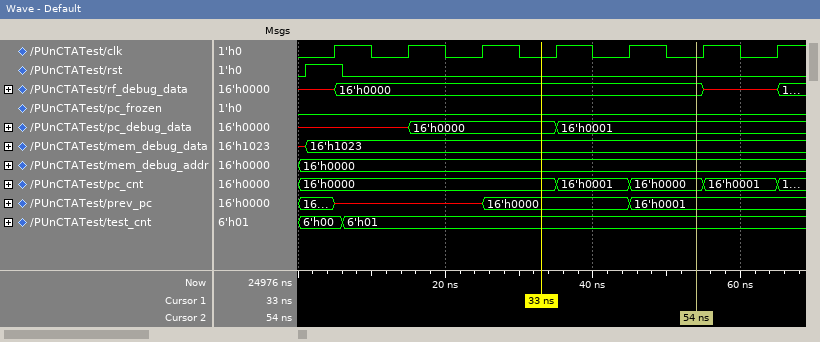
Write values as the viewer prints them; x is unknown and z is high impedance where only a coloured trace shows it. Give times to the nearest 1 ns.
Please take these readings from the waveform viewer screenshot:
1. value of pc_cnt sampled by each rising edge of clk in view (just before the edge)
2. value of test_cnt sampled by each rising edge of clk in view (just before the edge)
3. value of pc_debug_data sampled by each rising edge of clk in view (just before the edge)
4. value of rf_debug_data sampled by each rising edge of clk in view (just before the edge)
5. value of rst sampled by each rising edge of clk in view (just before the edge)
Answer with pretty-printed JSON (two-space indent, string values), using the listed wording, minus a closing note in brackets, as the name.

{
  "value of pc_cnt sampled by each rising edge of clk in view": "16'h0000, 16'h0000, 16'h0000, 16'h0000, 16'h0001, 16'h0000, 16'h0001",
  "value of test_cnt sampled by each rising edge of clk in view": "6'h00, 6'h01, 6'h01, 6'h01, 6'h01, 6'h01, 6'h01",
  "value of pc_debug_data sampled by each rising edge of clk in view": "x, x, 16'h0000, 16'h0000, 16'h0001, 16'h0001, 16'h0001",
  "value of rf_debug_data sampled by each rising edge of clk in view": "x, 16'h0000, 16'h0000, 16'h0000, 16'h0000, 16'h0000, x",
  "value of rst sampled by each rising edge of clk in view": "1 0 0 0 0 0 0"
}
